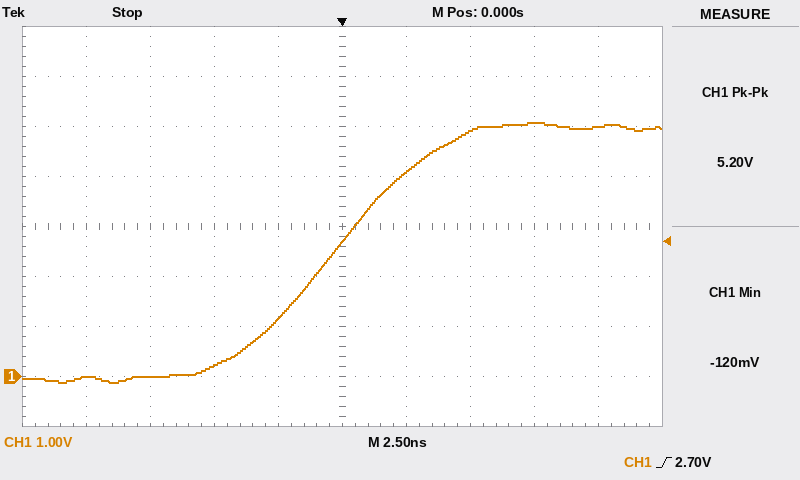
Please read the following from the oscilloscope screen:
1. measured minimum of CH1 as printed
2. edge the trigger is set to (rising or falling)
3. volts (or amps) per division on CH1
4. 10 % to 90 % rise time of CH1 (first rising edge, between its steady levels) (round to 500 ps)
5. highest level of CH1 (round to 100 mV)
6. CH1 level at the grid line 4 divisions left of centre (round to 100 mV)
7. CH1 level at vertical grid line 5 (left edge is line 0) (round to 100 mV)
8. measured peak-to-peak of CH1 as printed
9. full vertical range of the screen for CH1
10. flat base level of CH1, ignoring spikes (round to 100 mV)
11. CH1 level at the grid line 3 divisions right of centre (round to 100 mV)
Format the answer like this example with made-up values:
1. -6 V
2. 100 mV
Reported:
1. -120 mV
2. rising
3. 1 V
4. 7.5 ns
5. 5.1 V
6. 0.0 V
7. 2.7 V
8. 5.20 V
9. 8 V
10. 0.0 V
11. 5.1 V
